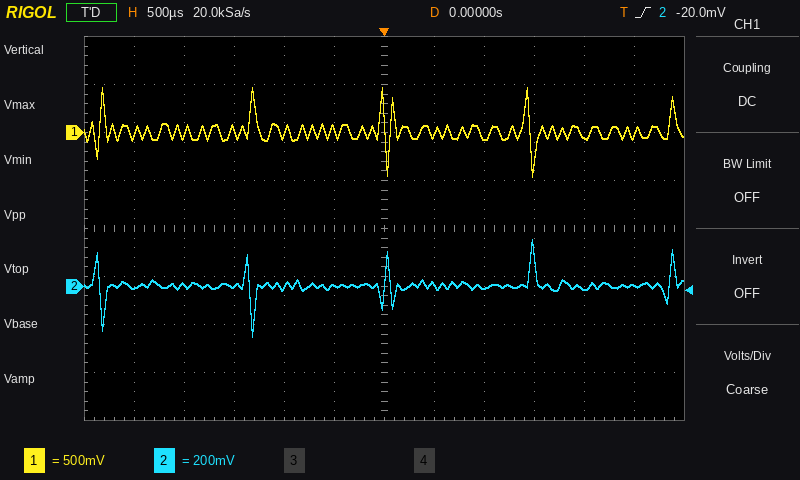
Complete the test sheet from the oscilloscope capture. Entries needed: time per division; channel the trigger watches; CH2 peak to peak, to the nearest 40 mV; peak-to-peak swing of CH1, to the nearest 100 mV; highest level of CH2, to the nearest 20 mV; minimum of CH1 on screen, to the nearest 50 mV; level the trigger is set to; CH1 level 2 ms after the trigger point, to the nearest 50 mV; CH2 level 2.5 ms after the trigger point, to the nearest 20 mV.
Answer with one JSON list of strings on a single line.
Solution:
["500 µs", "CH2", "400 mV", "900 mV", "200 mV", "-450 mV", "-20.0 mV", "-50 mV", "0 mV"]
